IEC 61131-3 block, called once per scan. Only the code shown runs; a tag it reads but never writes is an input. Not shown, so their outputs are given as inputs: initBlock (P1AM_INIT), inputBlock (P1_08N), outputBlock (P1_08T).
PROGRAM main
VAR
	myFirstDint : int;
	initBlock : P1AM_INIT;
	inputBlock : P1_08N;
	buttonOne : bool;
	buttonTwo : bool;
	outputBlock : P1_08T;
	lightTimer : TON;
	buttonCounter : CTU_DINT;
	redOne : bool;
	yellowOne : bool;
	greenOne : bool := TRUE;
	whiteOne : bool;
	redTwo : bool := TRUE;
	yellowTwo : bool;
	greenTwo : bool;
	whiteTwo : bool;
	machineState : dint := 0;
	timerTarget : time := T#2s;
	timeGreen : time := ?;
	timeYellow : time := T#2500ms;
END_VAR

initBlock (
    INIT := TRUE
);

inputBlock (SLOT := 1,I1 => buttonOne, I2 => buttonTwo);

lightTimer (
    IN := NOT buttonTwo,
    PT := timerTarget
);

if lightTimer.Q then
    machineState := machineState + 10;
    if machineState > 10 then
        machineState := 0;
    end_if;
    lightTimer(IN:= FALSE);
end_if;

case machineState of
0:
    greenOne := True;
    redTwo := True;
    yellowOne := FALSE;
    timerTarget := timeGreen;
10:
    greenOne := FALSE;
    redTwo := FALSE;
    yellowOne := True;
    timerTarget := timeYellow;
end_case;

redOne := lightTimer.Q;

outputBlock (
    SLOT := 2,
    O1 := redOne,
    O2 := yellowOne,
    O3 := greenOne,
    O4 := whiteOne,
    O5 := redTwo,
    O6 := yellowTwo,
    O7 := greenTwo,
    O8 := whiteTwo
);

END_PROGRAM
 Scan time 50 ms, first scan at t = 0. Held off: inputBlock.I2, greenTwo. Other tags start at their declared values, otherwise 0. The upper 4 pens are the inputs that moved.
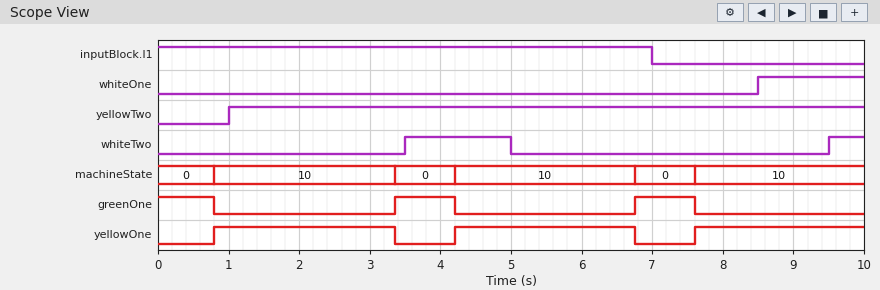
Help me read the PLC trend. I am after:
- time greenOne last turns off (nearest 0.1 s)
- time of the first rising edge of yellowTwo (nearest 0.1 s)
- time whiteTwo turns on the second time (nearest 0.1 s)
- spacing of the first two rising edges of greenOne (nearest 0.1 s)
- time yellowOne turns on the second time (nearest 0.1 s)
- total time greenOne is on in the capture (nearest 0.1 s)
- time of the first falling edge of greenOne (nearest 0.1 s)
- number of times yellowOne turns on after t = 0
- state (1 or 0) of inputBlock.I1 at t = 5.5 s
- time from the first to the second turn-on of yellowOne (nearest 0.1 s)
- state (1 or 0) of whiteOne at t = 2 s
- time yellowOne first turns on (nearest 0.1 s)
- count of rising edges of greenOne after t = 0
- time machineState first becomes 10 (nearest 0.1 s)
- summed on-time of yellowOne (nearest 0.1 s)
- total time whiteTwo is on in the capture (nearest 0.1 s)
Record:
7.6 s
1.0 s
9.5 s
3.4 s
4.2 s
2.5 s
0.8 s
3
1
3.4 s
0
0.8 s
2
0.8 s
7.5 s
2.0 s
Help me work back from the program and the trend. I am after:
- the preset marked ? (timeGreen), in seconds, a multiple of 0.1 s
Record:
0.8 s
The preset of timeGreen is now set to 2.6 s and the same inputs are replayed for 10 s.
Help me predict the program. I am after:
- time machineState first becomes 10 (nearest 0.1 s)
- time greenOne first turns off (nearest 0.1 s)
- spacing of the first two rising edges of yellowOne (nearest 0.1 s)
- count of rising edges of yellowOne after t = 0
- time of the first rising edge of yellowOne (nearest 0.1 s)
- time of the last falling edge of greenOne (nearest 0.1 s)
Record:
2.6 s
2.6 s
5.2 s
2
2.6 s
7.8 s
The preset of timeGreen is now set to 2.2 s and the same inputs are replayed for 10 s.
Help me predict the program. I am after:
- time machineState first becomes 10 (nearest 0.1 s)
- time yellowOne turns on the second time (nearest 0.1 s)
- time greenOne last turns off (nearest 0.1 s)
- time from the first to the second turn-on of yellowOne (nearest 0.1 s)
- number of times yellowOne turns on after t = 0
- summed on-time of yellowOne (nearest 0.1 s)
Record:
2.2 s
7.0 s
7.0 s
4.8 s
2
5.1 s
